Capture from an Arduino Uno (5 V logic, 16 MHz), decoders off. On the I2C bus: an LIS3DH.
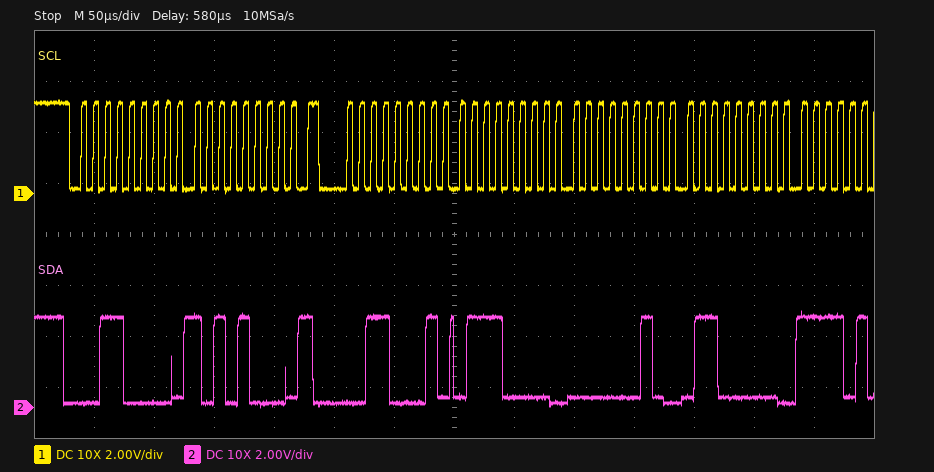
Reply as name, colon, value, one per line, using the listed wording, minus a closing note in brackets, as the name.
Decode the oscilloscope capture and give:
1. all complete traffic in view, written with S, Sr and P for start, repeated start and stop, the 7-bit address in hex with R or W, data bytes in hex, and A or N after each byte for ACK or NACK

all complete traffic in view, written with S, Sr and P for start, repeated start and stop, the 7-bit address in hex with R or W, data bytes in hex, and A or N after each byte for ACK or NACK: S 18W A A8 A Sr 18R A 70 A 02 A 60 A
